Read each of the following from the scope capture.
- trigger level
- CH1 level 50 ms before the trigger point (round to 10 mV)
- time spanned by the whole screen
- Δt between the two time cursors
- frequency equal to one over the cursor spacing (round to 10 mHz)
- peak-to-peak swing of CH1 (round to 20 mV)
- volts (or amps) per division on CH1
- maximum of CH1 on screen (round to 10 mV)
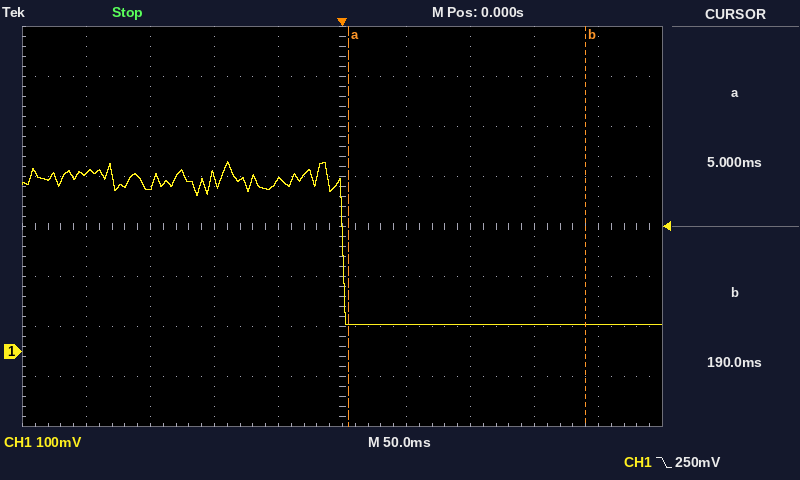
250 mV
340 mV
500 ms
185 ms
5.41 Hz
320 mV
100 mV
380 mV
